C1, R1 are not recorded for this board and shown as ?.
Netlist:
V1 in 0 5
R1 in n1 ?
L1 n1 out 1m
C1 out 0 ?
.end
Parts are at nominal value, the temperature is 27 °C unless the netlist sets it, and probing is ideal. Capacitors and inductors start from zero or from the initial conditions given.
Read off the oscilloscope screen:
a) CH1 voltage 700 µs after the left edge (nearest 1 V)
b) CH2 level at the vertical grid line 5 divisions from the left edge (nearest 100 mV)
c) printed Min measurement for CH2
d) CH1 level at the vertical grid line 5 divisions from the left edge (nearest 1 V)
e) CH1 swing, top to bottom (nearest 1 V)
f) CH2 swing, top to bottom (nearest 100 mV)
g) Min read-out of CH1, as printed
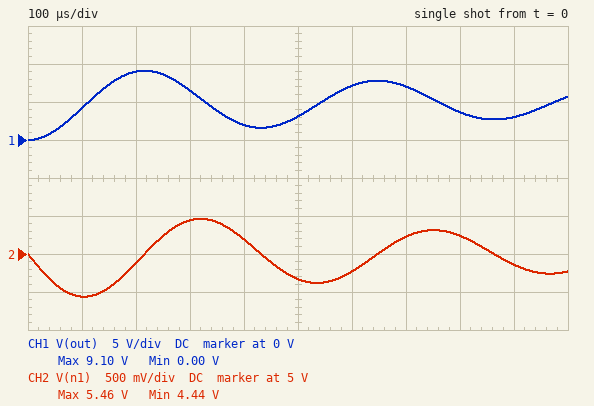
7 V
4.7 V
4.44 V
3 V
9 V
1.0 V
0.00 V
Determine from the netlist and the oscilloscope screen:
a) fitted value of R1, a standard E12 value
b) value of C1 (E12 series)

1.8 Ω
4.7 µF
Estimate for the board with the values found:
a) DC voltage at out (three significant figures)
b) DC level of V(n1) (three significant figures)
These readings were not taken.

5.00 V
5.00 V
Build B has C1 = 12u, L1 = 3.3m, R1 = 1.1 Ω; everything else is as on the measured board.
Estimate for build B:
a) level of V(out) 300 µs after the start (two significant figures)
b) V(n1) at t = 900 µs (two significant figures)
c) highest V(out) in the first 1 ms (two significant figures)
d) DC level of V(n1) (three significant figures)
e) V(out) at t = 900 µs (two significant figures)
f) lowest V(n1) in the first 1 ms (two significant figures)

4.5 V
5.3 V
9.5 V
5.00 V
6.0 V
4.7 V
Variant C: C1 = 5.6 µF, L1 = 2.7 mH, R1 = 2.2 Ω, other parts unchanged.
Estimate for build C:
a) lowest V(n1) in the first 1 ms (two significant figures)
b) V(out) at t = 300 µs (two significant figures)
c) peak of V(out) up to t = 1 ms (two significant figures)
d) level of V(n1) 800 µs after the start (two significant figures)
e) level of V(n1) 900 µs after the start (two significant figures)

4.5 V
8.2 V
9.3 V
4.9 V
4.7 V
